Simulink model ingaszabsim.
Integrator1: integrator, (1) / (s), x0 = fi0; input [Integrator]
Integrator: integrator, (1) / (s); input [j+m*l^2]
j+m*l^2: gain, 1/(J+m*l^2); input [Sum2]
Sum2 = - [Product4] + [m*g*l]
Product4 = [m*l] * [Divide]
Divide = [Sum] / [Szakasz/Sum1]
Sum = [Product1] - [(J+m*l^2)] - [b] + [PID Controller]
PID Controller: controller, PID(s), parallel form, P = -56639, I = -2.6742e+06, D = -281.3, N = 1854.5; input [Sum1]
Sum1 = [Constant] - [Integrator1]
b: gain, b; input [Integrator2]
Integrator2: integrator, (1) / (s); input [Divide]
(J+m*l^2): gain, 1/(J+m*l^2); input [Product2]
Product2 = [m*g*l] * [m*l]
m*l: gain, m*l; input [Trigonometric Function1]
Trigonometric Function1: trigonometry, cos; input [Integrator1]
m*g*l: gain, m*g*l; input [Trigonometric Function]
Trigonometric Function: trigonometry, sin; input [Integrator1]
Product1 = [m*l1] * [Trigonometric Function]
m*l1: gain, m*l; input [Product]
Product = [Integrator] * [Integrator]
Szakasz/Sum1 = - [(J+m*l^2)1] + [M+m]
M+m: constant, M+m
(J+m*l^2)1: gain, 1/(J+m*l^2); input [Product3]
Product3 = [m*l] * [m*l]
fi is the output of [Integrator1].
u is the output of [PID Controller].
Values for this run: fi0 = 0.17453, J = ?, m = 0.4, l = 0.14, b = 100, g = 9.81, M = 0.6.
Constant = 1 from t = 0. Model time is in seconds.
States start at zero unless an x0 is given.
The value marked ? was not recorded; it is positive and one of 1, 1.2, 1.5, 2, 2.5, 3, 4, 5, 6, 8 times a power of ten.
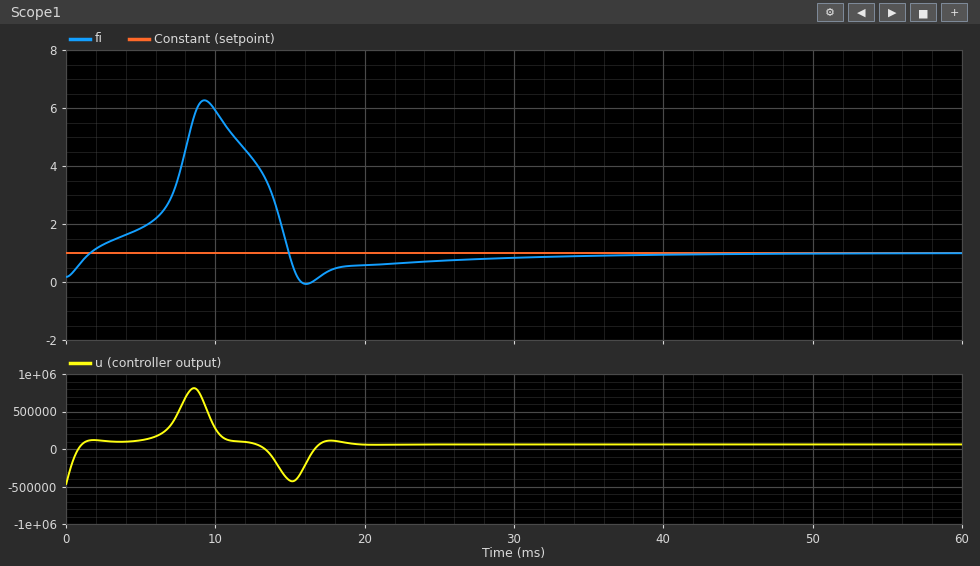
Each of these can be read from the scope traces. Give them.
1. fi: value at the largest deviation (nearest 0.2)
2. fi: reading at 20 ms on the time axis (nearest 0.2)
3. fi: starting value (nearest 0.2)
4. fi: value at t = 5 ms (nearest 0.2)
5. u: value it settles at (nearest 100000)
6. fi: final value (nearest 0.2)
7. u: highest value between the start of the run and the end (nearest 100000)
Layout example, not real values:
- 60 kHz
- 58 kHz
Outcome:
- 6.2
- 0.6
- 0.2
- 1.8
- 100000
- 1.0
- 800000
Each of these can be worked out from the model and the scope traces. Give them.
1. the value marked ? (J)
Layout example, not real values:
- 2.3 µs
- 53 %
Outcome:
- 0.008
